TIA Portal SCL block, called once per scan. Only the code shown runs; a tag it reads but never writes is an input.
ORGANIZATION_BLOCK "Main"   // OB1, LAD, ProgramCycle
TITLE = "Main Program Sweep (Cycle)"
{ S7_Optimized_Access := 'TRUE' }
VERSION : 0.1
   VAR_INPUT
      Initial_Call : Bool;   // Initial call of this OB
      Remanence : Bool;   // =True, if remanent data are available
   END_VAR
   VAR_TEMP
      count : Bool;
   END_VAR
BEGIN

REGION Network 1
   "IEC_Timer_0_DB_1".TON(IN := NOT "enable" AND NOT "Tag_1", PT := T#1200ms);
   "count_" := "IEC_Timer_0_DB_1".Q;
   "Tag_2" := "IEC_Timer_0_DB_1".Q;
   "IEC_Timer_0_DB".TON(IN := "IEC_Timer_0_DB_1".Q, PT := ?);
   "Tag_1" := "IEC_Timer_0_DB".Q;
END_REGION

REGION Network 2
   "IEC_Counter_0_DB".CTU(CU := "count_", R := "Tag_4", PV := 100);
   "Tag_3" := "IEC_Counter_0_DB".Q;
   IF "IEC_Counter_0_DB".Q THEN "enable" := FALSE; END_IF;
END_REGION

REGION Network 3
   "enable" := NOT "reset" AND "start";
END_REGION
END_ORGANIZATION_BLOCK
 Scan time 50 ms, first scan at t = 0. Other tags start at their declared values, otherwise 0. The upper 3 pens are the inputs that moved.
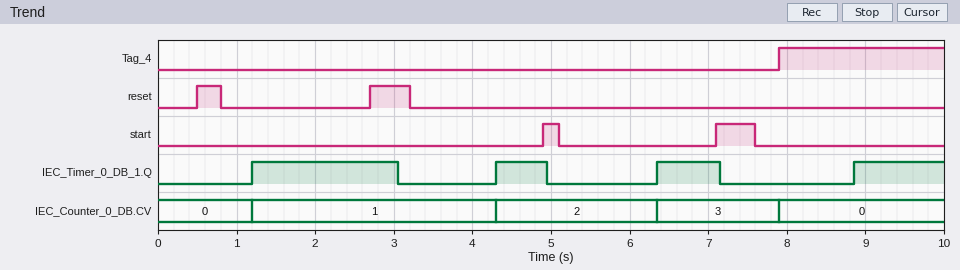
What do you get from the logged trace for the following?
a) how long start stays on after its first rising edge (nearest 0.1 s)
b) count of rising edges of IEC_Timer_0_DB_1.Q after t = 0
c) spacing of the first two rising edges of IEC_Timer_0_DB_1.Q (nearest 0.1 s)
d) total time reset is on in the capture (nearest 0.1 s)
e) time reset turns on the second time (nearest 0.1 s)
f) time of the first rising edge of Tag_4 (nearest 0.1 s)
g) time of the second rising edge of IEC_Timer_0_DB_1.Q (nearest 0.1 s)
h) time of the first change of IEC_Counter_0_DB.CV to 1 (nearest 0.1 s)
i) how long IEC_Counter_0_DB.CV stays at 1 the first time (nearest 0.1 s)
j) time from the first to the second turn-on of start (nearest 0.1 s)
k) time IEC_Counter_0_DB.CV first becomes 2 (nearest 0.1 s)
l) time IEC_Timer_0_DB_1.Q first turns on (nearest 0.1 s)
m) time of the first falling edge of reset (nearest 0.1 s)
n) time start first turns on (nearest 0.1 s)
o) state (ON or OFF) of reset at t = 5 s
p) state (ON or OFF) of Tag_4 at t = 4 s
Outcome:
0.2 s
4
3.1 s
0.8 s
2.7 s
7.9 s
4.3 s
1.2 s
3.1 s
2.2 s
4.3 s
1.2 s
0.8 s
4.9 s
OFF
OFF
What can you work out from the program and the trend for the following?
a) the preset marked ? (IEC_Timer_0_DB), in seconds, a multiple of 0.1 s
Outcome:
1.8 s
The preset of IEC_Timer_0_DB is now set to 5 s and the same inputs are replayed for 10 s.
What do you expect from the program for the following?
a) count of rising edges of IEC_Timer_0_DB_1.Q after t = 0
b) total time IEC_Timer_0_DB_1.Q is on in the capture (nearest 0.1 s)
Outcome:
3
5.7 s
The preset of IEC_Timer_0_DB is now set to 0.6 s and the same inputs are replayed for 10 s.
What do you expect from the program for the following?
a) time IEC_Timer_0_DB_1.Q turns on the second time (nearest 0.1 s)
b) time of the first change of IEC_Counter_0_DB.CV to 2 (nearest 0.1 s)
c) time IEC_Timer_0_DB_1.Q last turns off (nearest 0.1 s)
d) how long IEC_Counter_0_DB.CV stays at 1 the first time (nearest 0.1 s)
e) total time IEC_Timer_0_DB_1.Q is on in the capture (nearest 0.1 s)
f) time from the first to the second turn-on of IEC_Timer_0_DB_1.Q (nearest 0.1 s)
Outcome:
3.1 s
3.1 s
9.5 s
1.9 s
2.6 s
1.9 s
